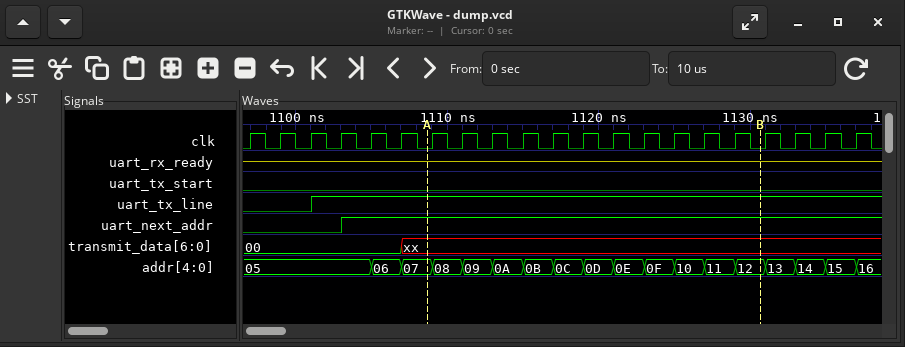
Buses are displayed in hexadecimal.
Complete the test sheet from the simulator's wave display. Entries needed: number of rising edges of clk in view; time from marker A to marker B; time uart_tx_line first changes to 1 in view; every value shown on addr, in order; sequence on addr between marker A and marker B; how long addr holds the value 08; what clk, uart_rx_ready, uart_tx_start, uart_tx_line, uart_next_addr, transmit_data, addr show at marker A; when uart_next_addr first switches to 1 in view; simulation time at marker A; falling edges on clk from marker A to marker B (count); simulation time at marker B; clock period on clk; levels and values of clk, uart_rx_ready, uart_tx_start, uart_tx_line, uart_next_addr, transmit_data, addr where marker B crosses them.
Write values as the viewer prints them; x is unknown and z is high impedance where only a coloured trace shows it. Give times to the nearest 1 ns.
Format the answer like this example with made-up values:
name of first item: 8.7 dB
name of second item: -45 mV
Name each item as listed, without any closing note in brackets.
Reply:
number of rising edges of clk in view: 21
time from marker A to marker B: 22 ns
time uart_tx_line first changes to 1 in view: 1101 ns
every value shown on addr, in order: 05, 06, 07, 08, 09, 0A, 0B, 0C, 0D, 0E, 0F, 10, 11, 12, 13, 14, 15, 16
sequence on addr between marker A and marker B: 07, 08, 09, 0A, 0B, 0C, 0D, 0E, 0F, 10, 11, 12
how long addr holds the value 08: 2 ns
what clk, uart_rx_ready, uart_tx_start, uart_tx_line, uart_next_addr, transmit_data, addr show at marker A: clk=0, uart_rx_ready=z, uart_tx_start=0, uart_tx_line=1, uart_next_addr=1, transmit_data=xx, addr=07
when uart_next_addr first switches to 1 in view: 1103 ns
simulation time at marker A: 1109 ns
falling edges on clk from marker A to marker B: 11
simulation time at marker B: 1131 ns
clock period on clk: 2 ns
levels and values of clk, uart_rx_ready, uart_tx_start, uart_tx_line, uart_next_addr, transmit_data, addr where marker B crosses them: clk=0, uart_rx_ready=z, uart_tx_start=0, uart_tx_line=1, uart_next_addr=1, transmit_data=xx, addr=12
